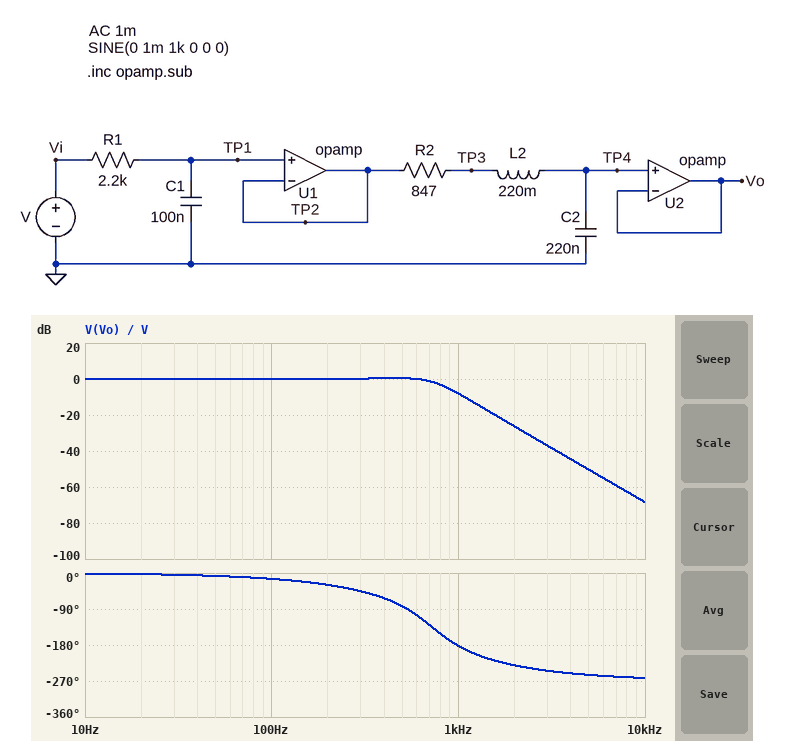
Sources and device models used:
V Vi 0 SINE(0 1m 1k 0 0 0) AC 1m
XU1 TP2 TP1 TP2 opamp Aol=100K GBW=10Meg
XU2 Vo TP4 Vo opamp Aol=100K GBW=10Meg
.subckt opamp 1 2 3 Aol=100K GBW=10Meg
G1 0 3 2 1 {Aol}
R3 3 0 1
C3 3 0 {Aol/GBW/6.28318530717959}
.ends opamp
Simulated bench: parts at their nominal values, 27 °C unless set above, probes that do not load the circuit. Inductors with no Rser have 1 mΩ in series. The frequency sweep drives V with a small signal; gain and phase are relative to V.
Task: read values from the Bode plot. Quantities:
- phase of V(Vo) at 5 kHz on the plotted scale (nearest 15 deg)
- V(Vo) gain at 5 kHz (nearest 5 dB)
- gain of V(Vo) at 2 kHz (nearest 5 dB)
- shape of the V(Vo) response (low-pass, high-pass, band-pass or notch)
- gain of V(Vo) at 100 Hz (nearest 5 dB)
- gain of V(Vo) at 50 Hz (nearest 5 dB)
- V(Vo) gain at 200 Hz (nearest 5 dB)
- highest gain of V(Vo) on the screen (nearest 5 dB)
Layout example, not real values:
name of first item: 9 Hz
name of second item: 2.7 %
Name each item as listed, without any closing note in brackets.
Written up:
phase of V(Vo) at 5 kHz on the plotted scale: -255 deg
V(Vo) gain at 5 kHz: -50 dB
gain of V(Vo) at 2 kHz: -25 dB
shape of the V(Vo) response: low-pass
gain of V(Vo) at 100 Hz: 0 dB
gain of V(Vo) at 50 Hz: 0 dB
V(Vo) gain at 200 Hz: 0 dB
highest gain of V(Vo) on the screen: 0 dB
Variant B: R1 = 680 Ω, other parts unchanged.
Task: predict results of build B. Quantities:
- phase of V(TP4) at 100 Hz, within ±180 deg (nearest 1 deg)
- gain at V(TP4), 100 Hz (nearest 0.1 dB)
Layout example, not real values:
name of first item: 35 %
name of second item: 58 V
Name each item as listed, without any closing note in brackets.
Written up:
phase of V(TP4) at 100 Hz, within ±180 deg: -9 deg
gain at V(TP4), 100 Hz: 0.1 dB
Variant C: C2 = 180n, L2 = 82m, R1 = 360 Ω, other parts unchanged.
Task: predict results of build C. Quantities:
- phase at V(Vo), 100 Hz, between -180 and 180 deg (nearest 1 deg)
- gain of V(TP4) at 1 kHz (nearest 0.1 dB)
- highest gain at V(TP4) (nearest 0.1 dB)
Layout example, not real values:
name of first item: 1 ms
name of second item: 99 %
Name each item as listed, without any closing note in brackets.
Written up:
phase at V(Vo), 100 Hz, between -180 and 180 deg: -7 deg
gain of V(TP4) at 1 kHz: -0.6 dB
highest gain at V(TP4): 0.1 dB
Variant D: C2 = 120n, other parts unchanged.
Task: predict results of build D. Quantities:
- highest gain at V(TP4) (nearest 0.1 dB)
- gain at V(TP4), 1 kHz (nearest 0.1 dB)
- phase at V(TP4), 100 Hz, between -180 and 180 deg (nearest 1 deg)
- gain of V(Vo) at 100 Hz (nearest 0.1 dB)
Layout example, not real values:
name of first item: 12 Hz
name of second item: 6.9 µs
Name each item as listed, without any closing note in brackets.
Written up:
highest gain at V(TP4): 0.8 dB
gain at V(TP4), 1 kHz: -0.8 dB
phase at V(TP4), 100 Hz, between -180 and 180 deg: -12 deg
gain of V(Vo) at 100 Hz: 0 dB
